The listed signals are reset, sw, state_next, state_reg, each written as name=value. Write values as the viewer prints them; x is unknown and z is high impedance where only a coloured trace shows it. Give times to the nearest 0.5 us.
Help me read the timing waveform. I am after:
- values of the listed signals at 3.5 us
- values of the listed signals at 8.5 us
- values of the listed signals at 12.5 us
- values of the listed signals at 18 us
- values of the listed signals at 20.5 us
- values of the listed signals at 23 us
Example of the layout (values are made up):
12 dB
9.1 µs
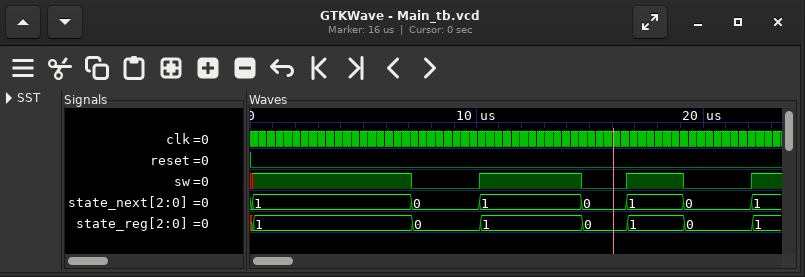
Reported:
reset=0, sw=1, state_next=1, state_reg=1
reset=0, sw=0, state_next=0, state_reg=0
reset=0, sw=1, state_next=1, state_reg=1
reset=0, sw=1, state_next=1, state_reg=1
reset=0, sw=0, state_next=0, state_reg=0
reset=0, sw=1, state_next=1, state_reg=1
